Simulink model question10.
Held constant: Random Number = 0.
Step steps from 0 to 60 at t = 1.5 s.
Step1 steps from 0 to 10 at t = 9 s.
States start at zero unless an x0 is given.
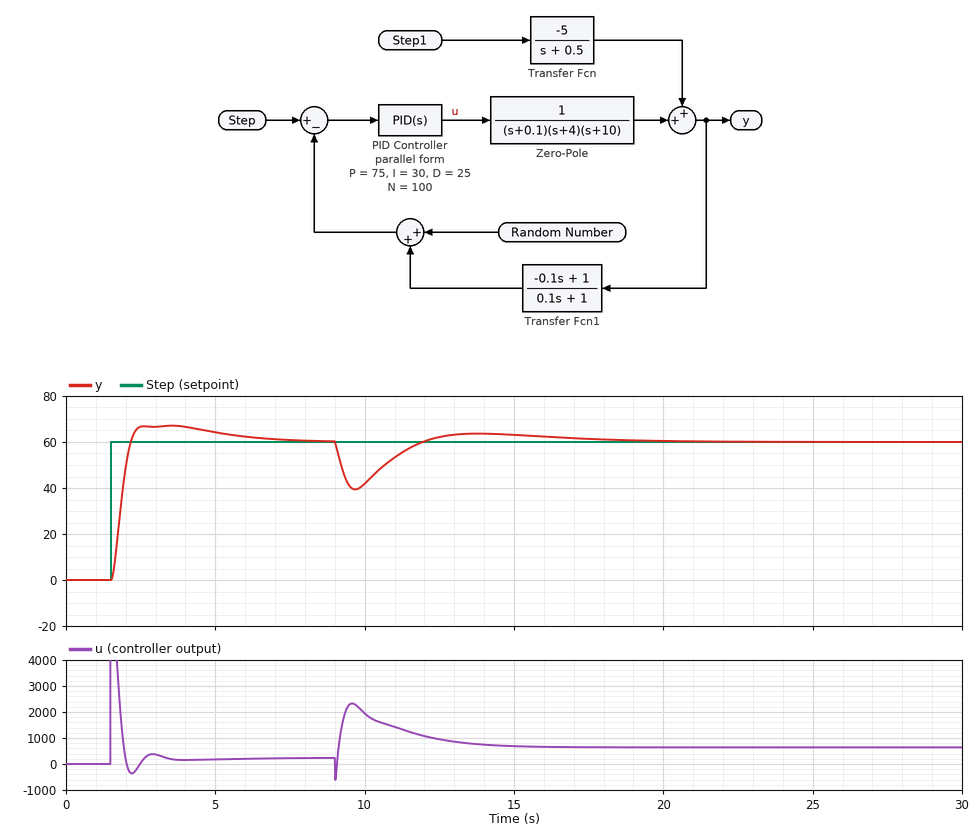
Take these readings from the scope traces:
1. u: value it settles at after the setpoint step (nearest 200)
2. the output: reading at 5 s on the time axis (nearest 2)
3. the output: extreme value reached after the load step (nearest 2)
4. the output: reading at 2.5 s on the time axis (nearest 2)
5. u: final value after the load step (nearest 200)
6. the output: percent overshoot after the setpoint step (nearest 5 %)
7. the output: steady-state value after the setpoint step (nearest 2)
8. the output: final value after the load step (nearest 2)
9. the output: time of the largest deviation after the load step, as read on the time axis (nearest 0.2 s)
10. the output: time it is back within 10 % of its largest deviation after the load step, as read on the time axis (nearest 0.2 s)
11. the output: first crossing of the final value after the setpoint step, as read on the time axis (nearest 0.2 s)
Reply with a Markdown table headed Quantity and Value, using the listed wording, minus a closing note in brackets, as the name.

| Quantity | Value |
|---|---|
| u: value it settles at after the setpoint step | 200 |
| the output: reading at 5 s on the time axis | 64 |
| the output: extreme value reached after the load step | 40 |
| the output: reading at 2.5 s on the time axis | 66 |
| u: final value after the load step | 600 |
| the output: percent overshoot after the setpoint step | 10 % |
| the output: steady-state value after the setpoint step | 60 |
| the output: final value after the load step | 60 |
| the output: time of the largest deviation after the load step, as read on the time axis | 9.6 s |
| the output: time it is back within 10 % of its largest deviation after the load step, as read on the time axis | 16.4 s |
| the output: first crossing of the final value after the setpoint step, as read on the time axis | 2.2 s |
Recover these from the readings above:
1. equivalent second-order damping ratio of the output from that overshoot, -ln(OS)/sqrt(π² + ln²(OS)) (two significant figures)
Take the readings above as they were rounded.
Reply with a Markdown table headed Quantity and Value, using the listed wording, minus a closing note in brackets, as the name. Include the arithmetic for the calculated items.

| Quantity | Value |
|---|---|
| equivalent second-order damping ratio of the output from that overshoot, -ln(OS)/sqrt(π² + ln²(OS)) | ln(0.1) = -2.303; 2.303 / sqrt(9.870 + 5.302) = 0.59 |
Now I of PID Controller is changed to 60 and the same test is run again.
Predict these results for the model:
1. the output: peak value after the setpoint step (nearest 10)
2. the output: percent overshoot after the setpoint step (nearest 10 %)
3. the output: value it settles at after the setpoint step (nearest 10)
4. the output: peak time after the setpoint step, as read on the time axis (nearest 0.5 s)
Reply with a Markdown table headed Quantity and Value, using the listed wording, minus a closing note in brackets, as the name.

| Quantity | Value |
|---|---|
| the output: peak value after the setpoint step | 80 |
| the output: percent overshoot after the setpoint step | 30 % |
| the output: value it settles at after the setpoint step | 60 |
| the output: peak time after the setpoint step, as read on the time axis | 3.0 s |
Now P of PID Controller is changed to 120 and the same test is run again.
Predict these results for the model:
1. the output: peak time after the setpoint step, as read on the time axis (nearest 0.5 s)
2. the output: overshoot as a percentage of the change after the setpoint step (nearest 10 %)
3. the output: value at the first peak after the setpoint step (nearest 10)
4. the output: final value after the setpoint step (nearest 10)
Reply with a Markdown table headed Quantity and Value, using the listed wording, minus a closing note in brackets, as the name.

| Quantity | Value |
|---|---|
| the output: peak time after the setpoint step, as read on the time axis | 2.5 s |
| the output: overshoot as a percentage of the change after the setpoint step | 40 % |
| the output: value at the first peak after the setpoint step | 80 |
| the output: final value after the setpoint step | 60 |
